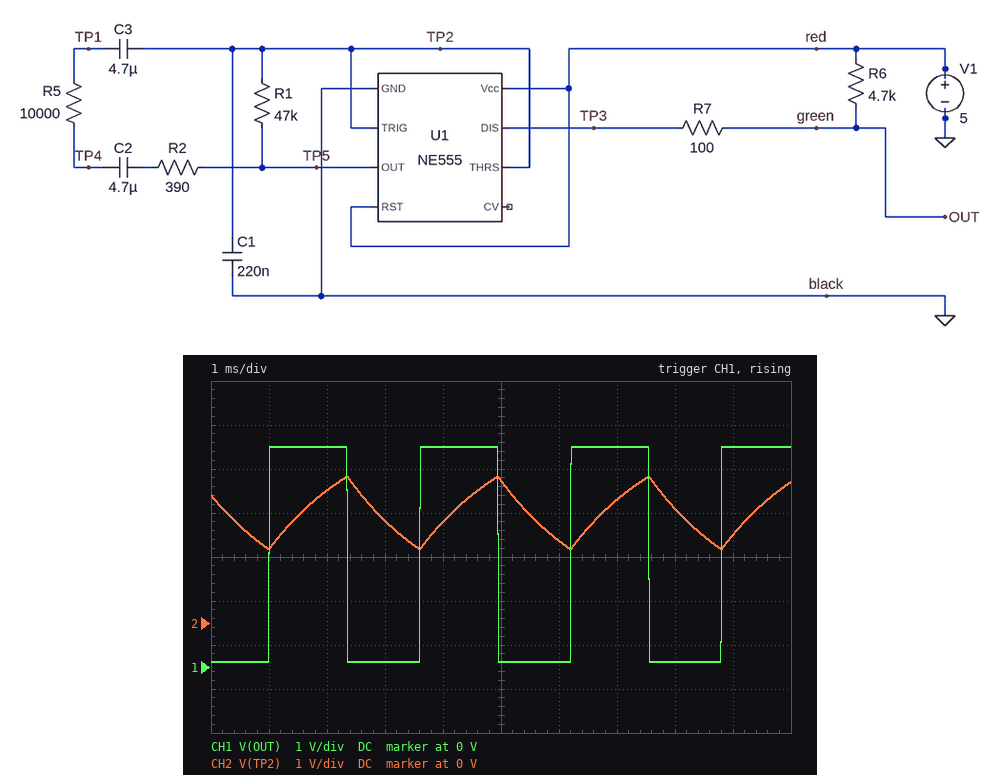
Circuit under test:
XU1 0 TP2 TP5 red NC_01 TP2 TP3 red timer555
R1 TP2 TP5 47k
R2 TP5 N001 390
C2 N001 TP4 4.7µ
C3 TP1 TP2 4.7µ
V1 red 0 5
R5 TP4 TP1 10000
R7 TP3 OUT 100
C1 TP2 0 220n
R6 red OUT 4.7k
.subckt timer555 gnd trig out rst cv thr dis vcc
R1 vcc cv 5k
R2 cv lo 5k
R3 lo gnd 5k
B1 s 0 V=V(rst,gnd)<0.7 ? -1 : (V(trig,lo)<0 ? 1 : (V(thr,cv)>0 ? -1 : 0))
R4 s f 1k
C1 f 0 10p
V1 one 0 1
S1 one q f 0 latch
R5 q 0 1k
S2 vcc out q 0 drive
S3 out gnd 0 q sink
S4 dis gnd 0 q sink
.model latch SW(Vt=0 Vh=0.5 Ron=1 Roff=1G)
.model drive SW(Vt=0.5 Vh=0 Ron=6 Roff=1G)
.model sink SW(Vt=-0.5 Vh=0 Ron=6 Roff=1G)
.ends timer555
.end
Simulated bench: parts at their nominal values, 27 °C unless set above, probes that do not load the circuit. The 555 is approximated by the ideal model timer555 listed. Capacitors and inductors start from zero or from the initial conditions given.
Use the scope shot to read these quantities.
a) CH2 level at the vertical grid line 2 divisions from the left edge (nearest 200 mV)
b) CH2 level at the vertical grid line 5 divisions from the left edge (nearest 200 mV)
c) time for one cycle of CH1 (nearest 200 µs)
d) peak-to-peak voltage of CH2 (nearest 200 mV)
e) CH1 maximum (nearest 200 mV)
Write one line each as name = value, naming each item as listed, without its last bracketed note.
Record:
CH2 level at the vertical grid line 2 divisions from the left edge = 3.0 V
CH2 level at the vertical grid line 5 divisions from the left edge = 3.2 V
time for one cycle of CH1 = 2.6 ms
peak-to-peak voltage of CH2 = 1.6 V
CH1 maximum = 5.0 V
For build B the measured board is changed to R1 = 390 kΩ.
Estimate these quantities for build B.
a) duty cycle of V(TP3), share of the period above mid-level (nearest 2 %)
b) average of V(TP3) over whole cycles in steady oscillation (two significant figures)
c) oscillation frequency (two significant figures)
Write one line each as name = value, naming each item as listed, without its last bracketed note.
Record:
duty cycle of V(TP3), share of the period above mid-level = 54 %
average of V(TP3) over whole cycles in steady oscillation = 2.7 V
oscillation frequency = 320 Hz
